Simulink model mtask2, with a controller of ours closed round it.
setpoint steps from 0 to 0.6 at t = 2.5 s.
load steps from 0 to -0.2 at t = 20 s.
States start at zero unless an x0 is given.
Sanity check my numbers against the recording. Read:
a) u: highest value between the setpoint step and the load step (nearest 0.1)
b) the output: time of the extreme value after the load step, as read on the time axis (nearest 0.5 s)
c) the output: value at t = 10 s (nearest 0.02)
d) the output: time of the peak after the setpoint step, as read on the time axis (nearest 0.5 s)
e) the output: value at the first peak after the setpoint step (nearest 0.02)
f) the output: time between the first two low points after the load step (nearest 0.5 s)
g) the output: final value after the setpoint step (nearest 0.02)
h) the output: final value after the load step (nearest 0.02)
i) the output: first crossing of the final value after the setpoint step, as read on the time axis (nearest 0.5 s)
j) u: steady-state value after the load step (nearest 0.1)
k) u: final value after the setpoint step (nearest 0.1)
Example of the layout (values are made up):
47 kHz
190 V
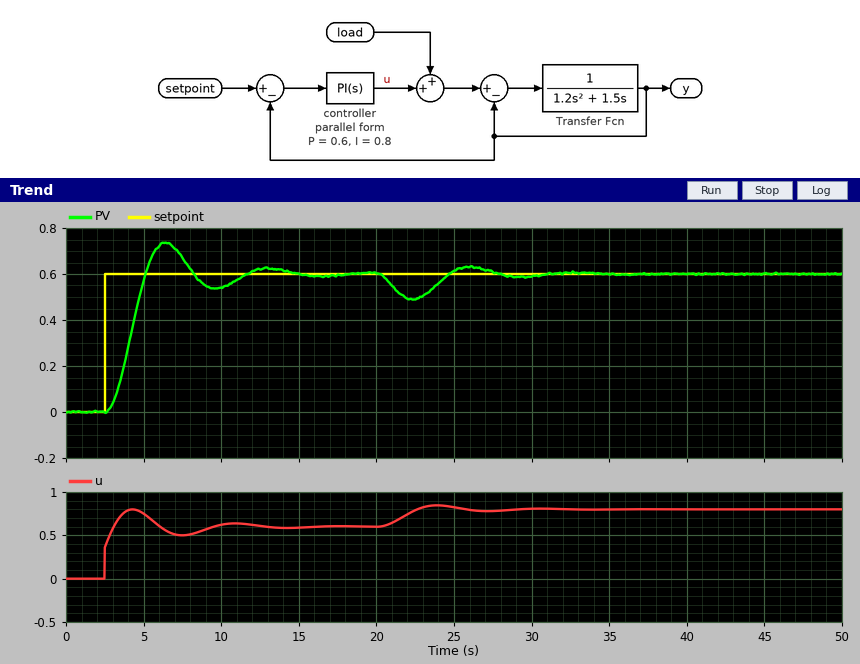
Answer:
0.8
22.5 s
0.54
6.5 s
0.74
7.0 s
0.60
0.60
5.0 s
0.8
0.6
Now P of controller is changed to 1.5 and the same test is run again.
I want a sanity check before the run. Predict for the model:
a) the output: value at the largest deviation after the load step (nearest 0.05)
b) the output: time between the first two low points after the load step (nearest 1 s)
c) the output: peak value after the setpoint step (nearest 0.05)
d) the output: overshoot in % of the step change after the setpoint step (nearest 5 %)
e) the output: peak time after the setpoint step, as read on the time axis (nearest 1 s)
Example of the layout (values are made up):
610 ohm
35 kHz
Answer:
0.50
5 s
0.65
10 %
5 s
